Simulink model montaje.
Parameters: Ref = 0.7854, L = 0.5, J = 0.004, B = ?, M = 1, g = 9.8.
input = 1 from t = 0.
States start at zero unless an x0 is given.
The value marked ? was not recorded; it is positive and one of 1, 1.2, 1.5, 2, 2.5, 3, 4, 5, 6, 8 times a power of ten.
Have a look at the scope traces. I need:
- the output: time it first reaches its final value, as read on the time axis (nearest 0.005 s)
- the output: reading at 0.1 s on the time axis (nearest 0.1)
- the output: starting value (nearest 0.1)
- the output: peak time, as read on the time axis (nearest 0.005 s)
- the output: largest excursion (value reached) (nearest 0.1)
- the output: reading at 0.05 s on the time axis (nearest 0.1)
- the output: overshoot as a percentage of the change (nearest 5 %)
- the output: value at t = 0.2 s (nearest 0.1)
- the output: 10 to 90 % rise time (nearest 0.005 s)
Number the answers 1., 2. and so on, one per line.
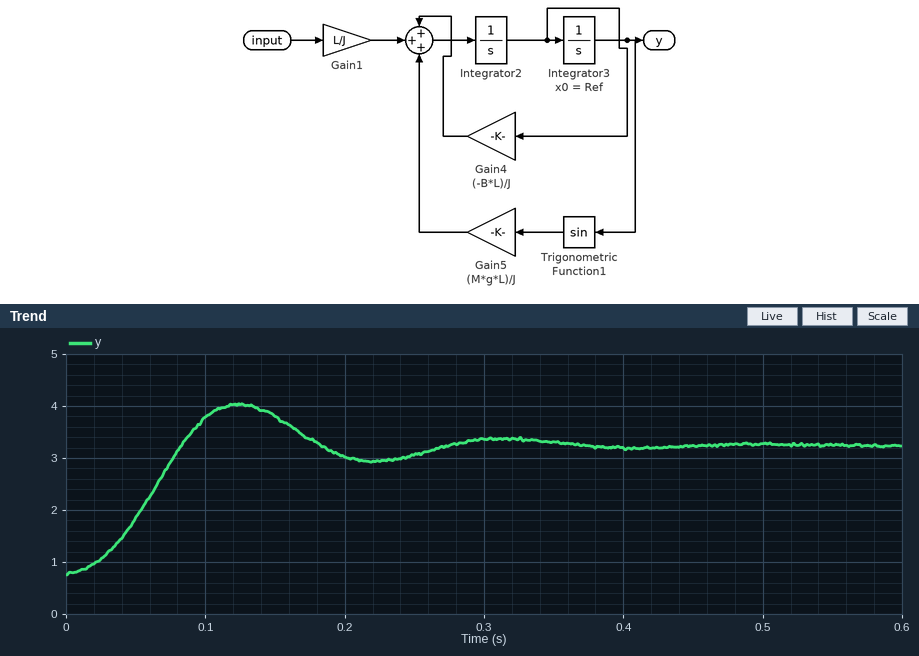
1. 0.085 s
2. 3.8
3. 0.8
4. 0.125 s
5. 4.0
6. 1.8
7. 30 %
8. 3.0
9. 0.055 s
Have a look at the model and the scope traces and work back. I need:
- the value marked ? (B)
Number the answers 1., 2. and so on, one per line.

1. 0.15
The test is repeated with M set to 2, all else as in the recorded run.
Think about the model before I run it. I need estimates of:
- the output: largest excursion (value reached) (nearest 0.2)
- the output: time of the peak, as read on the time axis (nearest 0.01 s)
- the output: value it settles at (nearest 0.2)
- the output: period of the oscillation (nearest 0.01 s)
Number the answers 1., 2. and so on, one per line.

1. 4.2
2. 0.09 s
3. 3.2
4. 0.13 s
